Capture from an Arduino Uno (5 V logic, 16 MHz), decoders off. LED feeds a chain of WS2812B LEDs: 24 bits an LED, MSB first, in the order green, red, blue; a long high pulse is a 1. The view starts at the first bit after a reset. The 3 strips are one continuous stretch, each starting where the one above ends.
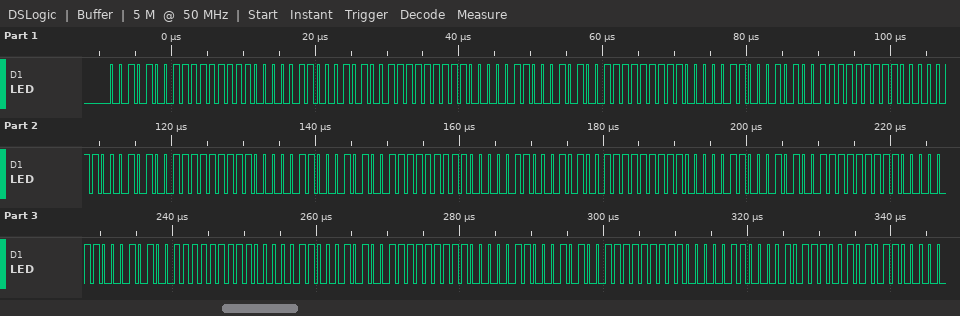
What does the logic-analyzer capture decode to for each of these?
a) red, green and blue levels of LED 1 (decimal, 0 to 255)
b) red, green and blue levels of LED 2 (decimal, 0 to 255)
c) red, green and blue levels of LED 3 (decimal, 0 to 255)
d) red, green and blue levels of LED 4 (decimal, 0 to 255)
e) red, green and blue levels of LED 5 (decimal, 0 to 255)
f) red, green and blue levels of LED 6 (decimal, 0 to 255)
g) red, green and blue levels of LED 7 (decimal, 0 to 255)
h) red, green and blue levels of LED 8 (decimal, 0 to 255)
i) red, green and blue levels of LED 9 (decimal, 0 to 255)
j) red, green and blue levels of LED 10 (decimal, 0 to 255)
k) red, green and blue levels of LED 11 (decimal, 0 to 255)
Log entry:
255, 41, 6
255, 41, 6
255, 41, 6
255, 41, 6
255, 41, 6
255, 41, 6
255, 41, 6
255, 41, 6
255, 41, 6
255, 41, 6
255, 41, 6
